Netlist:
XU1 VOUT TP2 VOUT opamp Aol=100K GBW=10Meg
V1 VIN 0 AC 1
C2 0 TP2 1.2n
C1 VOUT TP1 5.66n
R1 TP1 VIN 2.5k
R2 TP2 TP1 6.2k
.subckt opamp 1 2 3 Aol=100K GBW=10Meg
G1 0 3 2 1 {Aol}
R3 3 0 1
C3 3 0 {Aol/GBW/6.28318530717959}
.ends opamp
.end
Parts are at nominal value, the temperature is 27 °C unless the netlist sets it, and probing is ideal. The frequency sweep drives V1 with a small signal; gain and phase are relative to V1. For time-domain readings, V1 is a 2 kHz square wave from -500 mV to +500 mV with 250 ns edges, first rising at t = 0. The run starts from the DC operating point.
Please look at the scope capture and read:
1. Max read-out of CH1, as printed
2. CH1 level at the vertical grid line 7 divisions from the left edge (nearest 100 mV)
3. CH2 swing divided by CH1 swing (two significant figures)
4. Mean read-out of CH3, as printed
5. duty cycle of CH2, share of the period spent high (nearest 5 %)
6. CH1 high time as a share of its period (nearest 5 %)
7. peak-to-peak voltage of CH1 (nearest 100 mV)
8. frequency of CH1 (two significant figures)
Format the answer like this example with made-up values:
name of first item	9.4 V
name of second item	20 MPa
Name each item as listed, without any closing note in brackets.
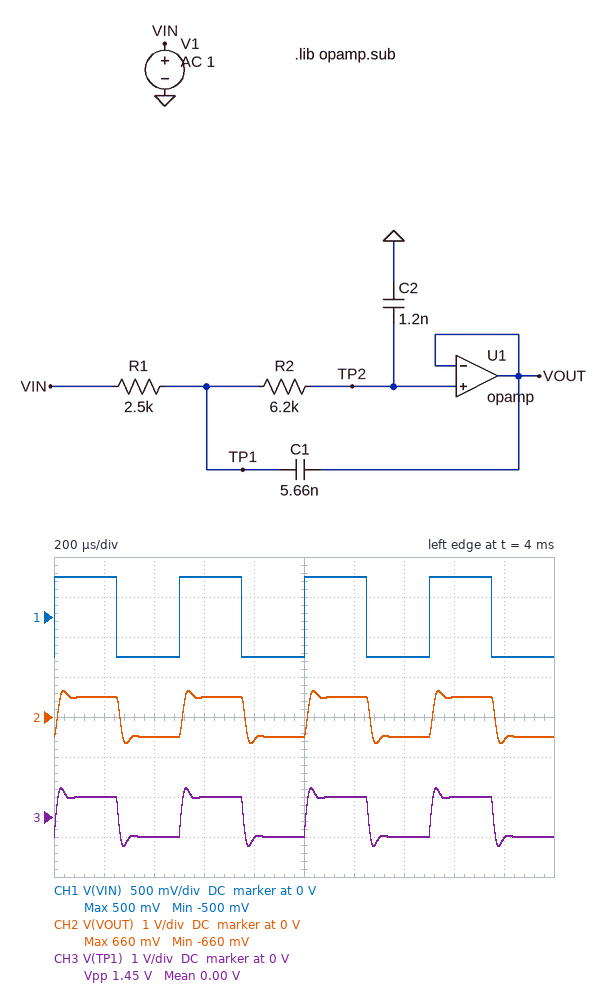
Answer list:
Max read-out of CH1, as printed	500 mV
CH1 level at the vertical grid line 7 divisions from the left edge	-500 mV
CH2 swing divided by CH1 swing	1.3
Mean read-out of CH3, as printed	0.00 V
duty cycle of CH2, share of the period spent high	50 %
CH1 high time as a share of its period	50 %
peak-to-peak voltage of CH1	1.0 V
frequency of CH1	2.0 kHz
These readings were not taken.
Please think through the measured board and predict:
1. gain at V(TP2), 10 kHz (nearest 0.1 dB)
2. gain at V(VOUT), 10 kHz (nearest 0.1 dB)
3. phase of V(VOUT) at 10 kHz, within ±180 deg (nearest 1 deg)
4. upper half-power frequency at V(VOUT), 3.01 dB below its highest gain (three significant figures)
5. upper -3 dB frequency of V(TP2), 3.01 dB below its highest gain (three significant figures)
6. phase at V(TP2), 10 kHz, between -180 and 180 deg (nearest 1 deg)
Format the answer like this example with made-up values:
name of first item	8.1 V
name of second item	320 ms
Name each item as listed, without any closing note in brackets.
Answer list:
gain at V(TP2), 10 kHz	1.1 dB
gain at V(VOUT), 10 kHz	1.1 dB
phase of V(VOUT) at 10 kHz, within ±180 deg	-48 deg
upper half-power frequency at V(VOUT), 3.01 dB below its highest gain	18.1 kHz
upper -3 dB frequency of V(TP2), 3.01 dB below its highest gain	18.1 kHz
phase at V(TP2), 10 kHz, between -180 and 180 deg	-48 deg
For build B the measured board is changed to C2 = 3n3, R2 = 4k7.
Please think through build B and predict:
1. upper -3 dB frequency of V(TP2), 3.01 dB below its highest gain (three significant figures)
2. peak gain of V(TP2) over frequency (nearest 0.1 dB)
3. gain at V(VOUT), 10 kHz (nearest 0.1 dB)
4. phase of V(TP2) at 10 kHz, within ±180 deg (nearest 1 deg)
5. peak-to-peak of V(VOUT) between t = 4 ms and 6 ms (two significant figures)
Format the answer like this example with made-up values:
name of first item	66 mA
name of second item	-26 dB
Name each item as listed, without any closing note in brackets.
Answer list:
upper -3 dB frequency of V(TP2), 3.01 dB below its highest gain	9.33 kHz
peak gain of V(TP2) over frequency	0 dB
gain at V(VOUT), 10 kHz	-3.5 dB
phase of V(TP2) at 10 kHz, within ±180 deg	-85 deg
peak-to-peak of V(VOUT) between t = 4 ms and 6 ms	1.0 V
